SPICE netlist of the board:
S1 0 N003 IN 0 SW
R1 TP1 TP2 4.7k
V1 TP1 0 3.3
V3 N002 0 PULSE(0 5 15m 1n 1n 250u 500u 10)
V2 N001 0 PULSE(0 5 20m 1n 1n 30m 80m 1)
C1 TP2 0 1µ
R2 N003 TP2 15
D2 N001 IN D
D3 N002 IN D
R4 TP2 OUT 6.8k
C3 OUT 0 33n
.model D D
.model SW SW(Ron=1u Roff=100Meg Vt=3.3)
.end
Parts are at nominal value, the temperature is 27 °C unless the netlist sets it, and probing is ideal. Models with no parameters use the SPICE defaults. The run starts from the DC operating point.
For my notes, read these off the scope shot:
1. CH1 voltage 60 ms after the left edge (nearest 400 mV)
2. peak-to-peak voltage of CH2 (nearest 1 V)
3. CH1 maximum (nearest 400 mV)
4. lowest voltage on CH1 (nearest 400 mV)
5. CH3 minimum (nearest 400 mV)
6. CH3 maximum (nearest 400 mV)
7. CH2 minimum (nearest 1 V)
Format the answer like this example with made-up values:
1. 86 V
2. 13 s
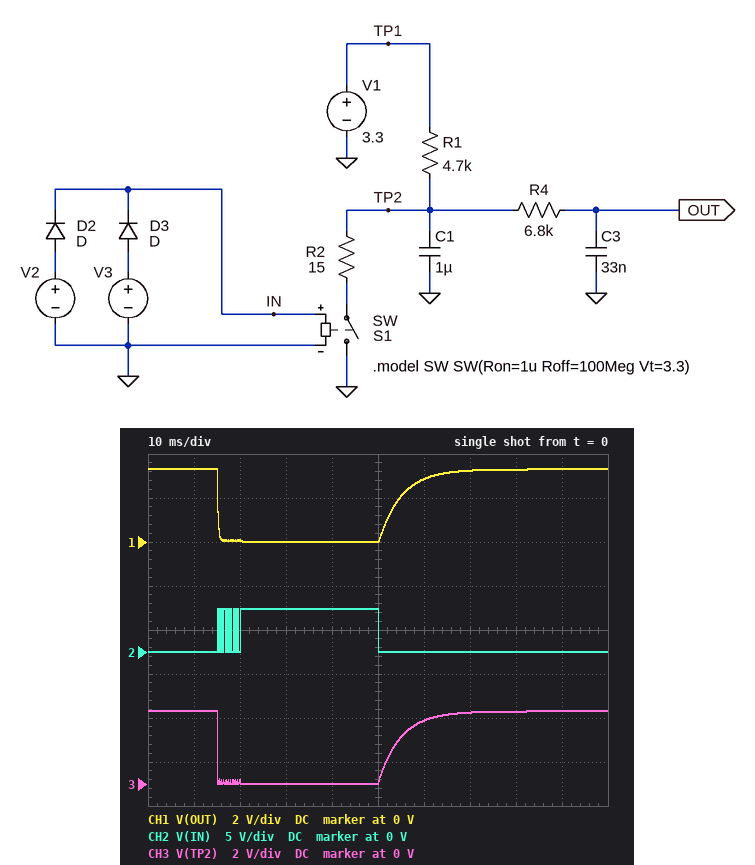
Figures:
1. 2.8 V
2. 5 V
3. 3.2 V
4. 0 V
5. 0 V
6. 3.2 V
7. 0 V
